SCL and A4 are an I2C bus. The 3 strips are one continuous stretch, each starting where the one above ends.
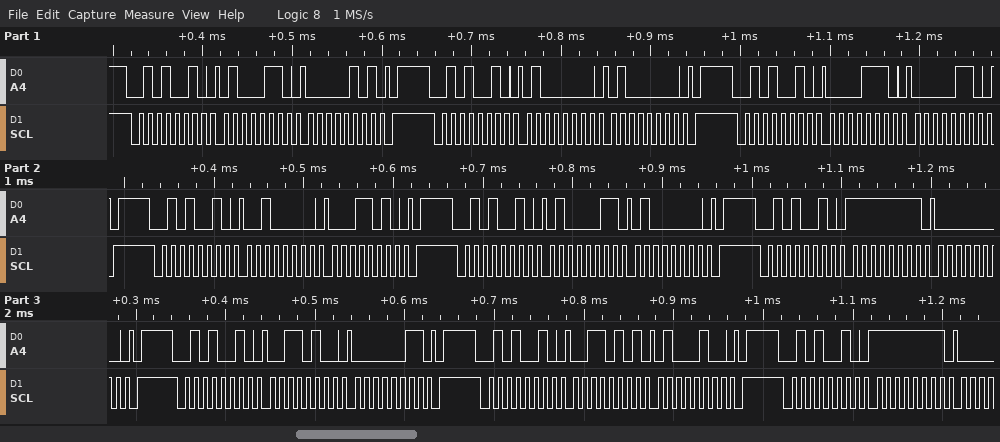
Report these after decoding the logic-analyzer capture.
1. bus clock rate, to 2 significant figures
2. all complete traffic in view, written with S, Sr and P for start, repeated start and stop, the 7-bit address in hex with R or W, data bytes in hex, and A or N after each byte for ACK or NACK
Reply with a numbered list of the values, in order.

1. 100 kHz
2. S 29W A 46 A 05 A P S 29W A 40 A 40 A P S 29W A 0E A 06 A P S 29W A 20 A 1A A P S 29W A 43 A 40 A P S 29W A FF A 00 A P S 29W A 34 A 03 A P S 29W A 35 A 44 A P S 29W A FF A
